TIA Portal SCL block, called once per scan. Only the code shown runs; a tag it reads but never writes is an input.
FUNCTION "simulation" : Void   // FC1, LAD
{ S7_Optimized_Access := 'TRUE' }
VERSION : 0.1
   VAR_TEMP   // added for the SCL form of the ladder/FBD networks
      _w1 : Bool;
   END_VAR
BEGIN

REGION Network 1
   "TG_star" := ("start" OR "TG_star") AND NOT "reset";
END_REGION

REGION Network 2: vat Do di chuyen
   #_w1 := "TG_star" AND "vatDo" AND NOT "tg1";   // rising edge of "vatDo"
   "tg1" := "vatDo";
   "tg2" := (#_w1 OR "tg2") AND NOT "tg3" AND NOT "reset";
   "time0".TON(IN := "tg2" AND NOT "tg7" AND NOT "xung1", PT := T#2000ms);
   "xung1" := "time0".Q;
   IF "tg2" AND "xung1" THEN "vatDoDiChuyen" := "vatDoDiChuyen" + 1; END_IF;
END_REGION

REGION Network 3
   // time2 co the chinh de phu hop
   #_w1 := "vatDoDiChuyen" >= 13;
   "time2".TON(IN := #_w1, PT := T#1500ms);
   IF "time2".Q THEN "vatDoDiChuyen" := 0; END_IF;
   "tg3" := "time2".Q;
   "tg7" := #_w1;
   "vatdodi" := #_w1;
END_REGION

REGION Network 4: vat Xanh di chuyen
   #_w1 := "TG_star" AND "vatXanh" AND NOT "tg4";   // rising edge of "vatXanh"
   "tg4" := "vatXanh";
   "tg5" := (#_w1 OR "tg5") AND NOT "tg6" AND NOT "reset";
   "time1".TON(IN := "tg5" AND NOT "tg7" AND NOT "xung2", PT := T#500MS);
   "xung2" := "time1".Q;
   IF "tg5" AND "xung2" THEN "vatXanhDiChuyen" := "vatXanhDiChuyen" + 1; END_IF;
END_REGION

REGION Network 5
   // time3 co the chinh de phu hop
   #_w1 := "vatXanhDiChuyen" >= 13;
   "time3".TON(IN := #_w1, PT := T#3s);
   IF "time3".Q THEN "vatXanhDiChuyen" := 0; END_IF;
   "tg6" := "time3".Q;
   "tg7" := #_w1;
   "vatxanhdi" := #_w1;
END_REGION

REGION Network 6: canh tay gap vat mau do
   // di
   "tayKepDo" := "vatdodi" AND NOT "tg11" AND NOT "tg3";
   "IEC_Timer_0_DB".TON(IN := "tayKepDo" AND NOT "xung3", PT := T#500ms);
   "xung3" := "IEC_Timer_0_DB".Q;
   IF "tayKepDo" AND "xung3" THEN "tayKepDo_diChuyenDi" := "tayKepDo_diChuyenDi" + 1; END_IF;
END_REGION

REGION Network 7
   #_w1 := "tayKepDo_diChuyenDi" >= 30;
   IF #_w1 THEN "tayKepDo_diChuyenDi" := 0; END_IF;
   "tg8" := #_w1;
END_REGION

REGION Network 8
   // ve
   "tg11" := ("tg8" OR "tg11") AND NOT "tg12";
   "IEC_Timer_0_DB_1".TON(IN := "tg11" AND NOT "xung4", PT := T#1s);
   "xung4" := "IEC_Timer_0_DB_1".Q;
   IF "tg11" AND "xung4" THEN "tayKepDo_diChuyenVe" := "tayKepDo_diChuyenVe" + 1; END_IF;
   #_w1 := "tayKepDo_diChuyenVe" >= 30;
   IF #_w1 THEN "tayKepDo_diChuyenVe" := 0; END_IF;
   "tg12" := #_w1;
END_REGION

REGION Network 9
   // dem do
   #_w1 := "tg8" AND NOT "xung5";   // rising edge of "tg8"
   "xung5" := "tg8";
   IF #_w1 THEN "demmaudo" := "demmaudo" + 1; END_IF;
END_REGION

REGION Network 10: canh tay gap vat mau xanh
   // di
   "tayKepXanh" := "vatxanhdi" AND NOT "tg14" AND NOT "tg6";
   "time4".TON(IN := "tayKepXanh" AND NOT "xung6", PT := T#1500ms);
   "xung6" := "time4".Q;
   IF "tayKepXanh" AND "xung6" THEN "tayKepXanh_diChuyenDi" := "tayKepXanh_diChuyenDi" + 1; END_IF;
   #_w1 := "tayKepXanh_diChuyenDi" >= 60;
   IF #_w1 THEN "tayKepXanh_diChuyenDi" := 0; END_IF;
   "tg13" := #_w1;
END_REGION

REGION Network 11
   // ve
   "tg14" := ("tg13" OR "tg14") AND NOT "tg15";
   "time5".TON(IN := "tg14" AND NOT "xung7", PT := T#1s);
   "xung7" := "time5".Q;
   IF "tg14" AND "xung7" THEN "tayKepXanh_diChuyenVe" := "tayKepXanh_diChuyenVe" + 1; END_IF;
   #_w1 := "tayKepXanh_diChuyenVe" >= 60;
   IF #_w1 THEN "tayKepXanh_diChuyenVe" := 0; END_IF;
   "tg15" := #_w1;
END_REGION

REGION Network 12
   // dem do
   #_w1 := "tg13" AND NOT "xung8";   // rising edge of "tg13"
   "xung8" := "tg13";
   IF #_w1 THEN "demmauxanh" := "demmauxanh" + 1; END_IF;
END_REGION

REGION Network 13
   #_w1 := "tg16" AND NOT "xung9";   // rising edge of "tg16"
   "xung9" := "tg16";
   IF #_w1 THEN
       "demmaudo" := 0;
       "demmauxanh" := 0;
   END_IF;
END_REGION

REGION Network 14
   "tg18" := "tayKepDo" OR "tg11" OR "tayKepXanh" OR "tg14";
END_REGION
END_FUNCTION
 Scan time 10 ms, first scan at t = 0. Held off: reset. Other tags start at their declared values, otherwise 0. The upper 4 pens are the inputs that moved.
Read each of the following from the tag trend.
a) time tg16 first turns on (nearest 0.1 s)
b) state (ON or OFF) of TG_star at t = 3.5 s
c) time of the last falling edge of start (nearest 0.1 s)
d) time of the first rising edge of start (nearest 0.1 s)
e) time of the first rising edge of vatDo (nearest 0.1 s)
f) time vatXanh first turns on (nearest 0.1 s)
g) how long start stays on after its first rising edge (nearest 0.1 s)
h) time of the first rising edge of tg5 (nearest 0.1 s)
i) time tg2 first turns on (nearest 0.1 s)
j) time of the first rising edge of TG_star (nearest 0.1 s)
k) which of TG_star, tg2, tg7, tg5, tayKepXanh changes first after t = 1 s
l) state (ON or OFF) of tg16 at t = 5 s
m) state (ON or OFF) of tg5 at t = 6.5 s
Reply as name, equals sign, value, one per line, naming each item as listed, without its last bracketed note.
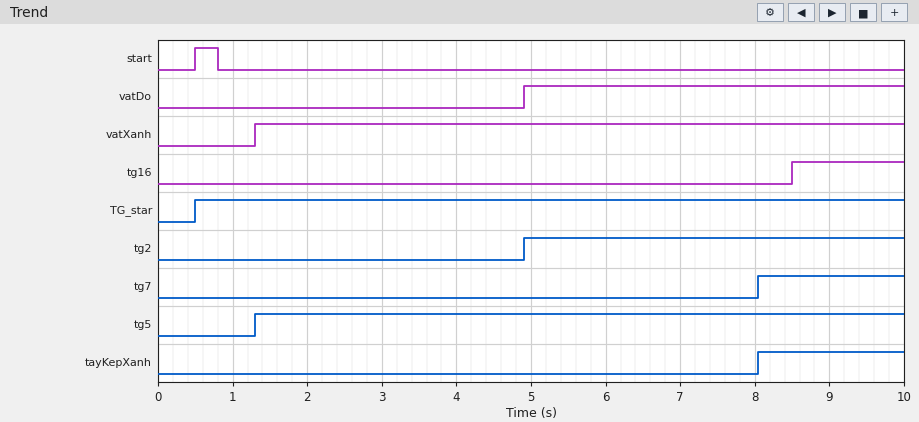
time tg16 first turns on = 8.5 s
state (ON or OFF) of TG_star at t = 3.5 s = ON
time of the last falling edge of start = 0.8 s
time of the first rising edge of start = 0.5 s
time of the first rising edge of vatDo = 4.9 s
time vatXanh first turns on = 1.3 s
how long start stays on after its first rising edge = 0.3 s
time of the first rising edge of tg5 = 1.3 s
time tg2 first turns on = 4.9 s
time of the first rising edge of TG_star = 0.5 s
which of TG_star, tg2, tg7, tg5, tayKepXanh changes first after t = 1 s = tg5
state (ON or OFF) of tg16 at t = 5 s = OFF
state (ON or OFF) of tg5 at t = 6.5 s = ON
